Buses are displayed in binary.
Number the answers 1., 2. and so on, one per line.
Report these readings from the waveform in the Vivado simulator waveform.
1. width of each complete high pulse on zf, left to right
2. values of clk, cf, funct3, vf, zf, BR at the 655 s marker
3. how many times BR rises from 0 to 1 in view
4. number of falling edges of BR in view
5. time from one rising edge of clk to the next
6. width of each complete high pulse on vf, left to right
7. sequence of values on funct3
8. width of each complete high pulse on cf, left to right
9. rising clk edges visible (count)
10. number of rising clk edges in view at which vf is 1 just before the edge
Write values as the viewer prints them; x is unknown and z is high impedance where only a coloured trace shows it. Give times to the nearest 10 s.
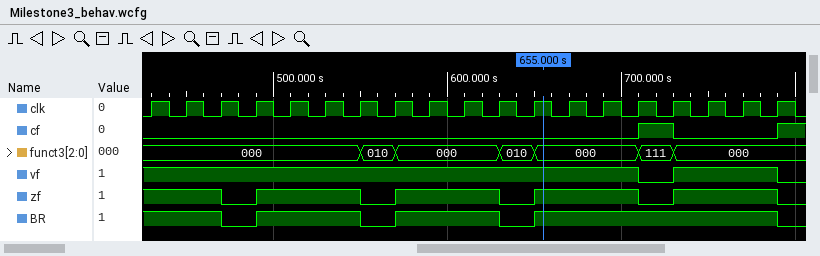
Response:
1. 60 s, 60 s, 60 s, 60 s
2. clk=1, cf=0, funct3=000, vf=1, zf=1, BR=1
3. 3
4. 4
5. 20 s
6. 60 s
7. 000, 010, 000, 010, 000, 111, 000
8. 20 s
9. 19
10. 18
